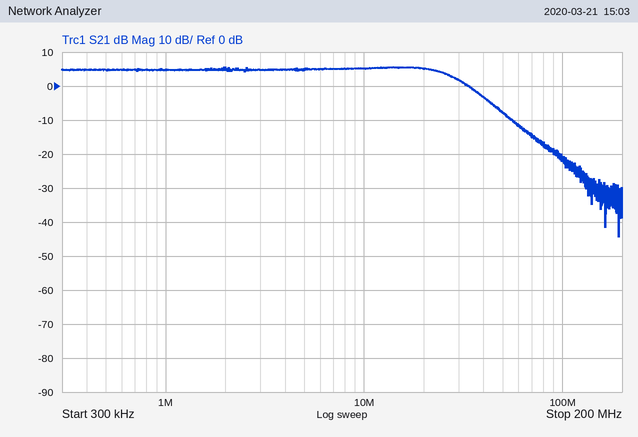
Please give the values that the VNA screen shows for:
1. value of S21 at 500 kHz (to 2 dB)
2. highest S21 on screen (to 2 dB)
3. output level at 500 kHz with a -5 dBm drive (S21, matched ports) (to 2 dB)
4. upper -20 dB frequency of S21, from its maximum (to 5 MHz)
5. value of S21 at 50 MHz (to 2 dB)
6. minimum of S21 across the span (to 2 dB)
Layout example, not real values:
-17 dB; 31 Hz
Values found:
4 dB; 6 dB; 0 dBm; 70 MHz; -8 dB; -44 dB
